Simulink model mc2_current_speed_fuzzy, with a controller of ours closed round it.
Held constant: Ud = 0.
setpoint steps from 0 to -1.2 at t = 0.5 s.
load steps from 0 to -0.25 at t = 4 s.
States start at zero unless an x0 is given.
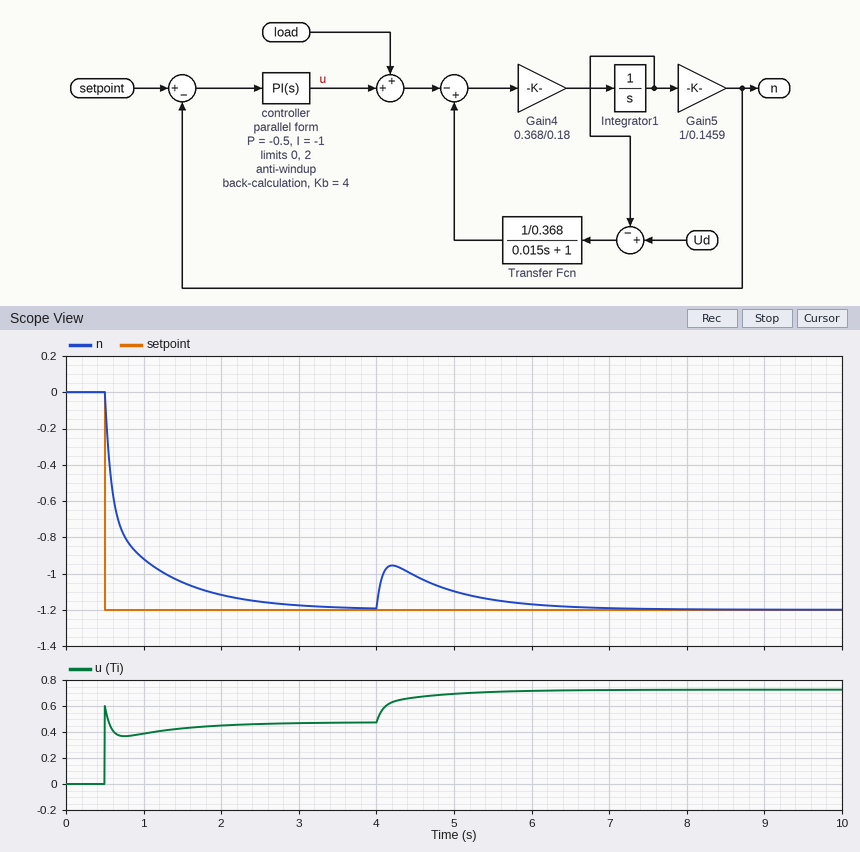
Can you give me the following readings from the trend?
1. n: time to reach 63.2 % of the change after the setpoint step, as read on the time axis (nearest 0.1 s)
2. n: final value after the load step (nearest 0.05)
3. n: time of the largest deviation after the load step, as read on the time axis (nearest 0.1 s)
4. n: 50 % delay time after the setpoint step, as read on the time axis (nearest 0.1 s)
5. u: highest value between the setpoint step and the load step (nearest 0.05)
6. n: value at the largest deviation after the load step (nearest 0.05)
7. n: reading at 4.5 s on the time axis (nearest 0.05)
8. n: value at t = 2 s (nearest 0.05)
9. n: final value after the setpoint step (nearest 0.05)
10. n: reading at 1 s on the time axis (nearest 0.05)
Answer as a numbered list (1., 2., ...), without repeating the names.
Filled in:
1. 0.7 s
2. -1.20
3. 4.2 s
4. 0.6 s
5. 0.60
6. -0.95
7. -1.00
8. -1.10
9. -1.20
10. -0.90
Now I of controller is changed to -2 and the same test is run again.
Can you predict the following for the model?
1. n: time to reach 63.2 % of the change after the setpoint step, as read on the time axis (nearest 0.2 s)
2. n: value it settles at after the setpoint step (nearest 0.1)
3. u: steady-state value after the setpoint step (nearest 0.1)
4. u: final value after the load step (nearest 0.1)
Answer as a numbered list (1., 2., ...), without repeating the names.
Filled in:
1. 0.6 s
2. -1.2
3. 0.5
4. 0.7
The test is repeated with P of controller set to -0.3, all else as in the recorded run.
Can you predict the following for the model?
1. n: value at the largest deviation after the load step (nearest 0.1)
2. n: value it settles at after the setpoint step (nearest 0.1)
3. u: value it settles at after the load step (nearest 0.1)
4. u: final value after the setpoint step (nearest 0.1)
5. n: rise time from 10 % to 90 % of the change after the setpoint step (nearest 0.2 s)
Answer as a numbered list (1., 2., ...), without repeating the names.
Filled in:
1. -0.9
2. -1.2
3. 0.7
4. 0.5
5. 1.0 s
